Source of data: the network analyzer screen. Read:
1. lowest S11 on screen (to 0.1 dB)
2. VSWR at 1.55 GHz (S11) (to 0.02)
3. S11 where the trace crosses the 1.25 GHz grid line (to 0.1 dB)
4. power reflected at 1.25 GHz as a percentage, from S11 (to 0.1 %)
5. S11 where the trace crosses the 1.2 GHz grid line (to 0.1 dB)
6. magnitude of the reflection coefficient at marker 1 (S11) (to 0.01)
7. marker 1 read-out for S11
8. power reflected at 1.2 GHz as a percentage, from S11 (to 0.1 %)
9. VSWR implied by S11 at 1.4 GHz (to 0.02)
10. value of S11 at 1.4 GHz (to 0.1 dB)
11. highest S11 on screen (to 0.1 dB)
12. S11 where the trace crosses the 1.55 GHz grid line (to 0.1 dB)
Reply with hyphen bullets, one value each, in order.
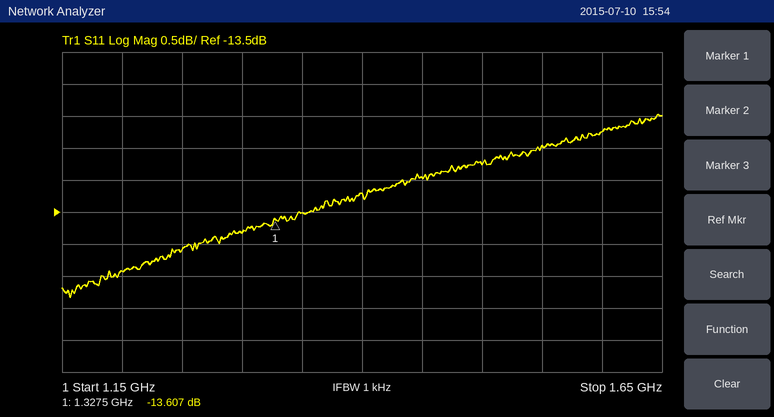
- -14.8 dB
- 1.62
- -14.1 dB
- 3.9 %
- -14.4 dB
- 0.21
- -13.607 dB
- 3.6 %
- 1.56
- -13.2 dB
- -12.0 dB
- -12.5 dB
